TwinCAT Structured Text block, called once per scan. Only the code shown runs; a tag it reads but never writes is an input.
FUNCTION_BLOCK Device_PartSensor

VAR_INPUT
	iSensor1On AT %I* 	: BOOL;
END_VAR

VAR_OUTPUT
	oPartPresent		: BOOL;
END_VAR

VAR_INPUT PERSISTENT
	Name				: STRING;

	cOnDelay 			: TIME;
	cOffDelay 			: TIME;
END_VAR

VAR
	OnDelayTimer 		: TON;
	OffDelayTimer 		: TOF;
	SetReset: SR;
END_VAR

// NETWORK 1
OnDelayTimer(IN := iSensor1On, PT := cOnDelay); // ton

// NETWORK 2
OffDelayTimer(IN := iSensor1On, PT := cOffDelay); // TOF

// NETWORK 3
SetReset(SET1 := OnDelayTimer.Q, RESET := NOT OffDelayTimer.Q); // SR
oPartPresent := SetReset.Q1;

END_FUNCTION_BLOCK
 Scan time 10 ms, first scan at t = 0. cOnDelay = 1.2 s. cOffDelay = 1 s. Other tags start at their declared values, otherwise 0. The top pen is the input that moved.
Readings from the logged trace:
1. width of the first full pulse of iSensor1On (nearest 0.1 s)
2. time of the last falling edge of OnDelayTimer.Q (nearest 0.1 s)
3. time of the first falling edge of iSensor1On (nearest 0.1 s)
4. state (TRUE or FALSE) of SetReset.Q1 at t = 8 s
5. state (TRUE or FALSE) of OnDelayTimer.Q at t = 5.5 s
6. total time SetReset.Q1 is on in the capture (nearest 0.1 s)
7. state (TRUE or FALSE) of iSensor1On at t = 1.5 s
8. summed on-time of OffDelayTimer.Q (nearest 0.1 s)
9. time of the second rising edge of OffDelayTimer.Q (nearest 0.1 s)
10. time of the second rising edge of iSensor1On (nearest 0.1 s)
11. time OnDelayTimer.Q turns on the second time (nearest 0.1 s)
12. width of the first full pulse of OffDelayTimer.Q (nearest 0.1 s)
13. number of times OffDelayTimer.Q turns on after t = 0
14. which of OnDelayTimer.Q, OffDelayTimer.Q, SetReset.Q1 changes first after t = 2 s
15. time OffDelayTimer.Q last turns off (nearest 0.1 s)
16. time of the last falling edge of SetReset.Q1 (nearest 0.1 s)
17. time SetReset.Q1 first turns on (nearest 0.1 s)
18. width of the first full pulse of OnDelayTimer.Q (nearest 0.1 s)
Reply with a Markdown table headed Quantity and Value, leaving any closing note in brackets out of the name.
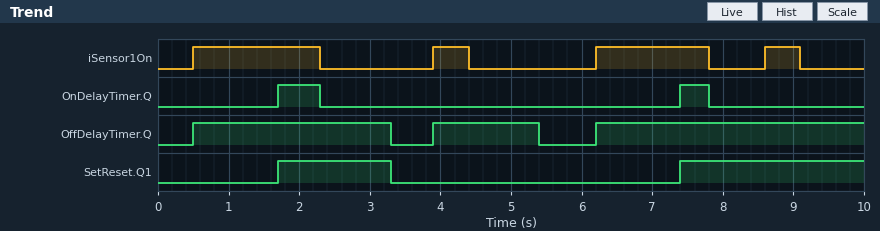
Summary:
| Quantity | Value |
|---|---|
| width of the first full pulse of iSensor1On | 1.8 s |
| time of the last falling edge of OnDelayTimer.Q | 7.8 s |
| time of the first falling edge of iSensor1On | 2.3 s |
| state (TRUE or FALSE) of SetReset.Q1 at t = 8 s | TRUE |
| state (TRUE or FALSE) of OnDelayTimer.Q at t = 5.5 s | FALSE |
| total time SetReset.Q1 is on in the capture | 4.2 s |
| state (TRUE or FALSE) of iSensor1On at t = 1.5 s | TRUE |
| summed on-time of OffDelayTimer.Q | 8.1 s |
| time of the second rising edge of OffDelayTimer.Q | 3.9 s |
| time of the second rising edge of iSensor1On | 3.9 s |
| time OnDelayTimer.Q turns on the second time | 7.4 s |
| width of the first full pulse of OffDelayTimer.Q | 2.8 s |
| number of times OffDelayTimer.Q turns on after t = 0 | 3 |
| which of OnDelayTimer.Q, OffDelayTimer.Q, SetReset.Q1 changes first after t = 2 s | OnDelayTimer.Q |
| time OffDelayTimer.Q last turns off | 5.4 s |
| time of the last falling edge of SetReset.Q1 | 3.3 s |
| time SetReset.Q1 first turns on | 1.7 s |
| width of the first full pulse of OnDelayTimer.Q | 0.6 s |
